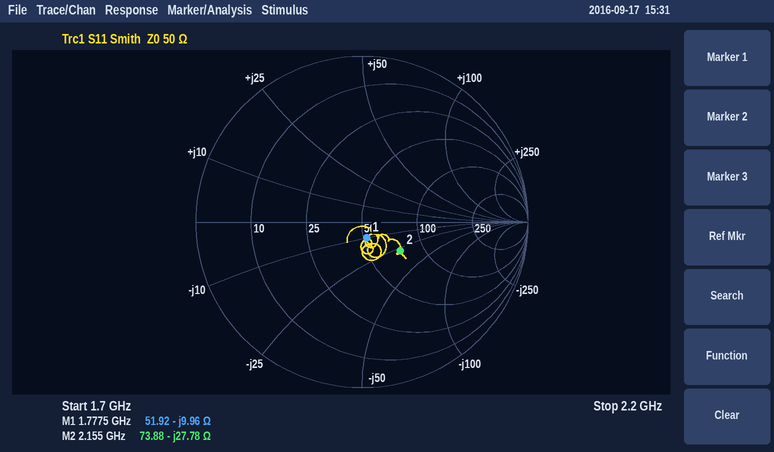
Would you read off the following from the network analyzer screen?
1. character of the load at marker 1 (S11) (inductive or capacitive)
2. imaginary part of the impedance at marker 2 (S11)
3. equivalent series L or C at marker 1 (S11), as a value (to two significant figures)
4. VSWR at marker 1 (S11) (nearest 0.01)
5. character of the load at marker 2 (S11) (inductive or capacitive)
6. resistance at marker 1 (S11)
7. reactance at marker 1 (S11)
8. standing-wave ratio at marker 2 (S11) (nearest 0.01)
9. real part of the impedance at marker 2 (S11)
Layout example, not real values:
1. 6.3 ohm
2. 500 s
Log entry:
1. capacitive
2. -27.78 Ω
3. 9.0 pF
4. 1.22
5. capacitive
6. 51.92 Ω
7. -9.96 Ω
8. 1.81
9. 73.88 Ω
